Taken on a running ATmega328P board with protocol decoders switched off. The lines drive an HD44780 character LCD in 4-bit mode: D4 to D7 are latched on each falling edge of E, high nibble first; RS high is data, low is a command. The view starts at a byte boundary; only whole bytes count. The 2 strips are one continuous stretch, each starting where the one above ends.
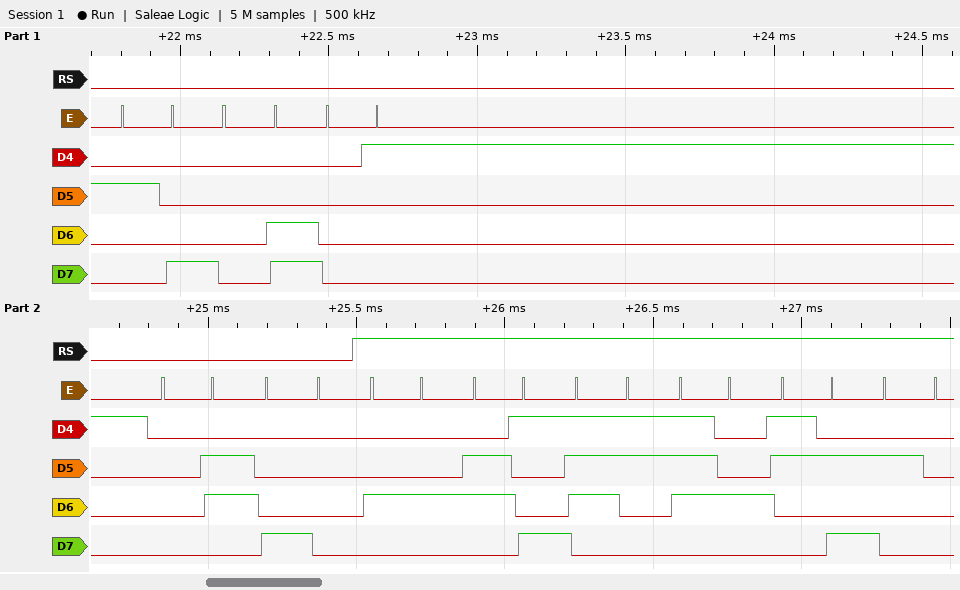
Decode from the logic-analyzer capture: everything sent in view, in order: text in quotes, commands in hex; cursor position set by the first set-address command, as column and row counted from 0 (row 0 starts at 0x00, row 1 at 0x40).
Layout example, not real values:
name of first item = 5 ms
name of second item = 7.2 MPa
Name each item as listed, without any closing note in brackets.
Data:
everything sent in view, in order: text in quotes, commands in hex = 0x28 0x0C 0x01 0x06 0x80 "Dist: "
cursor position set by the first set-address command, as column and row counted from 0 = column 0, row 0
